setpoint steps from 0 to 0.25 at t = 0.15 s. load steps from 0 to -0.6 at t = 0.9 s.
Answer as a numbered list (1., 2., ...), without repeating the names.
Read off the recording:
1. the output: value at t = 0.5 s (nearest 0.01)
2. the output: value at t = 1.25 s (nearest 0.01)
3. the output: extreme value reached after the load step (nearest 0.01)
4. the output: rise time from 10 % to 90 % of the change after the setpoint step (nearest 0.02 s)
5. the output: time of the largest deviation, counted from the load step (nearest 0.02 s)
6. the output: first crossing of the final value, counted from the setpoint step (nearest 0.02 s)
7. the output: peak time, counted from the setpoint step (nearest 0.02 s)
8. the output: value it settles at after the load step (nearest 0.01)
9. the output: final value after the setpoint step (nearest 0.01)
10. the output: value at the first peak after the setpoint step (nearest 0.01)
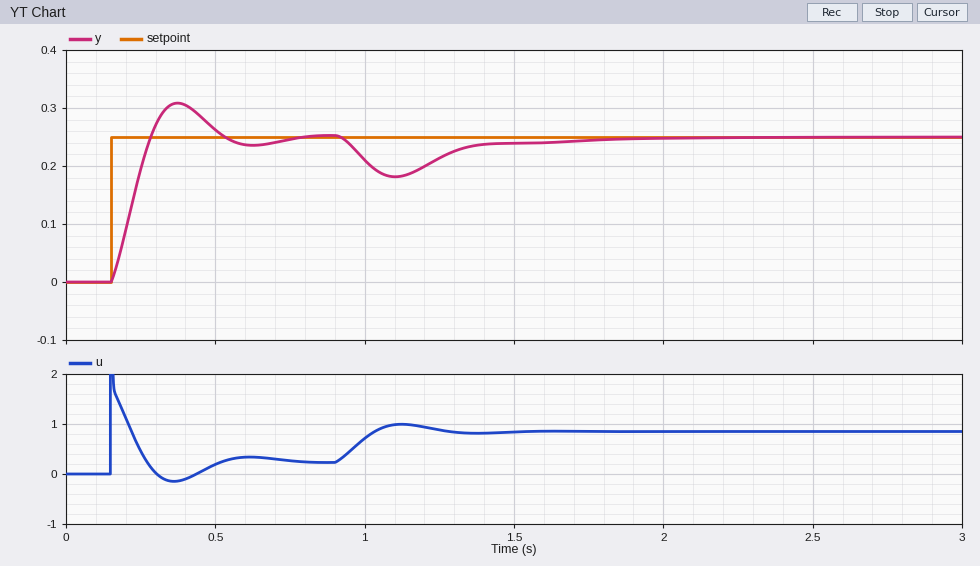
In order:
1. 0.26
2. 0.21
3. 0.18
4. 0.10 s
5. 0.20 s
6. 0.14 s
7. 0.22 s
8. 0.25
9. 0.25
10. 0.31
